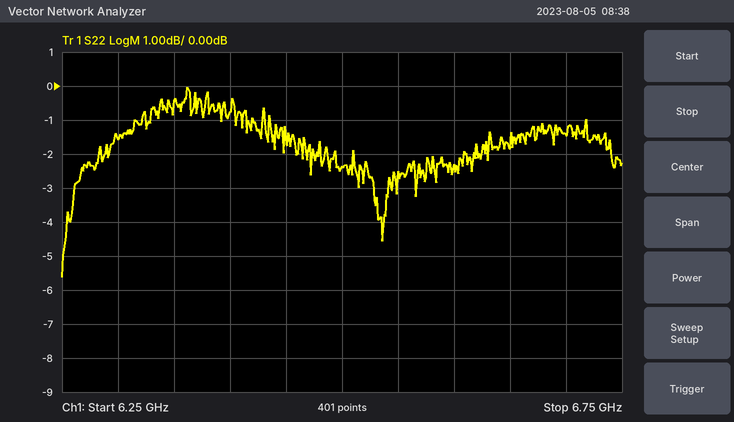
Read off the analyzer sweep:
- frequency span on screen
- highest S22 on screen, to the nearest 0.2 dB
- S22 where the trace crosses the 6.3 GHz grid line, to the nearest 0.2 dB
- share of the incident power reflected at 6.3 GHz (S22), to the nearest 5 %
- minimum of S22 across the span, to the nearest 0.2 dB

500 MHz
0.0 dB
-1.6 dB
70 %
-5.6 dB
